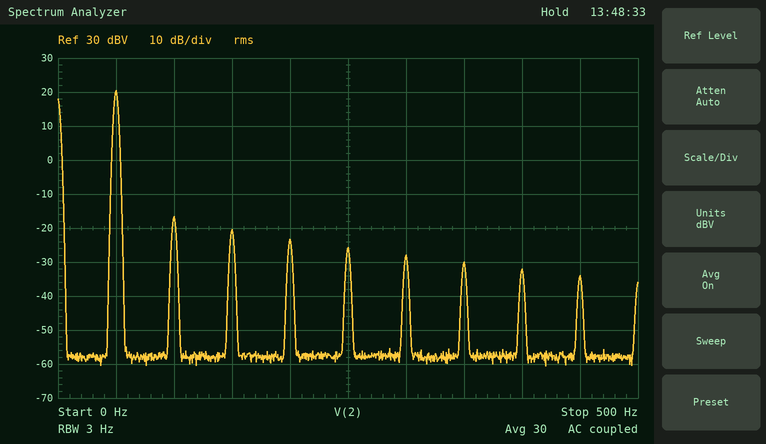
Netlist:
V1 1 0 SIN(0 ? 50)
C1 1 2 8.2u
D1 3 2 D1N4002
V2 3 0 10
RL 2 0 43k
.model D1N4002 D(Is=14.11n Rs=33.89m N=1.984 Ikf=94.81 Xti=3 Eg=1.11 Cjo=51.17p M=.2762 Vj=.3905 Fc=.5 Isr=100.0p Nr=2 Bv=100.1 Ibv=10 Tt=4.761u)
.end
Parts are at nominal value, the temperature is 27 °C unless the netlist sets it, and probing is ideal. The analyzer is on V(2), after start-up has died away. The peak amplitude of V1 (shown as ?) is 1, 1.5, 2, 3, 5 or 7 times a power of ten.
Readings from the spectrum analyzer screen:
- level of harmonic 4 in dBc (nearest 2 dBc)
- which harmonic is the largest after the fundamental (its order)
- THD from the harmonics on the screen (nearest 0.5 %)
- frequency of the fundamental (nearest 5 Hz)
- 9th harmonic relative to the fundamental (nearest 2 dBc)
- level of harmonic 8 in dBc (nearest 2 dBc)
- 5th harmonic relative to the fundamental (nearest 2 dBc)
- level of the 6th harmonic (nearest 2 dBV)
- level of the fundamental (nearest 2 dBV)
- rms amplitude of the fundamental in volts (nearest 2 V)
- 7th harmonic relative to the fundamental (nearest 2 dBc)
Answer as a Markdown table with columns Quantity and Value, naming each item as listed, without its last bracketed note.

| Quantity | Value |
|---|---|
| level of harmonic 4 in dBc | -44 dBc |
| which harmonic is the largest after the fundamental | 2 |
| THD from the harmonics on the screen | 2.0 % |
| frequency of the fundamental | 50 Hz |
| 9th harmonic relative to the fundamental | -54 dBc |
| level of harmonic 8 in dBc | -52 dBc |
| 5th harmonic relative to the fundamental | -46 dBc |
| level of the 6th harmonic | -28 dBV |
| level of the fundamental | 20 dBV |
| rms amplitude of the fundamental in volts | 10 V |
| 7th harmonic relative to the fundamental | -50 dBc |
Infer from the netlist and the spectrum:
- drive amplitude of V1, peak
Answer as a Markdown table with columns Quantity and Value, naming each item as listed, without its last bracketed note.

| Quantity | Value |
|---|---|
| drive amplitude of V1, peak | 15 V |
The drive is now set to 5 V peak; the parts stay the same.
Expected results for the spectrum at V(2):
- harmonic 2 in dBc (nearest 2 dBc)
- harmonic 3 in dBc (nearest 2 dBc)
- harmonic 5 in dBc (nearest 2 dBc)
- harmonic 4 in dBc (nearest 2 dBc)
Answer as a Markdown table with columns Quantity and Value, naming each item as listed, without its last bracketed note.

| Quantity | Value |
|---|---|
| harmonic 2 in dBc | -32 dBc |
| harmonic 3 in dBc | -36 dBc |
| harmonic 5 in dBc | -42 dBc |
| harmonic 4 in dBc | -40 dBc |
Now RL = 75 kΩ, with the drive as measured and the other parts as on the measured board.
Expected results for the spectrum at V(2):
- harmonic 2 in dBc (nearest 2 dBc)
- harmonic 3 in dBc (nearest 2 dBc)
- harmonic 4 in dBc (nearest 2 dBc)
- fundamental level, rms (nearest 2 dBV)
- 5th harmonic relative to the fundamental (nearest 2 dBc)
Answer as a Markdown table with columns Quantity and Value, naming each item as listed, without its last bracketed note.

| Quantity | Value |
|---|---|
| harmonic 2 in dBc | -42 dBc |
| harmonic 3 in dBc | -46 dBc |
| harmonic 4 in dBc | -48 dBc |
| fundamental level, rms | 20 dBV |
| 5th harmonic relative to the fundamental | -50 dBc |
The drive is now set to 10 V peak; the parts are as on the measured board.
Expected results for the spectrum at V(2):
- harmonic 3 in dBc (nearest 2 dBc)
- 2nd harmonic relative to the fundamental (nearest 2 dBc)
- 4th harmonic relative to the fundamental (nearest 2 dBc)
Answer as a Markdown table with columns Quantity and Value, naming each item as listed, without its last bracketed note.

| Quantity | Value |
|---|---|
| harmonic 3 in dBc | -40 dBc |
| 2nd harmonic relative to the fundamental | -36 dBc |
| 4th harmonic relative to the fundamental | -42 dBc |
